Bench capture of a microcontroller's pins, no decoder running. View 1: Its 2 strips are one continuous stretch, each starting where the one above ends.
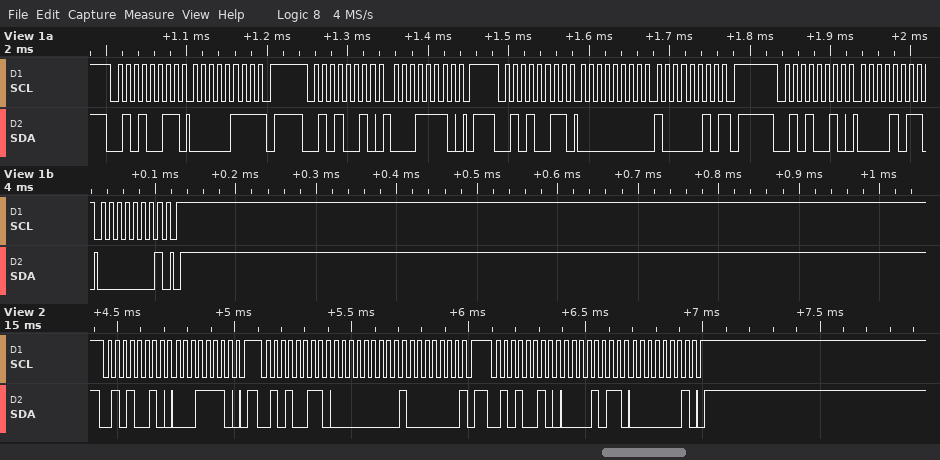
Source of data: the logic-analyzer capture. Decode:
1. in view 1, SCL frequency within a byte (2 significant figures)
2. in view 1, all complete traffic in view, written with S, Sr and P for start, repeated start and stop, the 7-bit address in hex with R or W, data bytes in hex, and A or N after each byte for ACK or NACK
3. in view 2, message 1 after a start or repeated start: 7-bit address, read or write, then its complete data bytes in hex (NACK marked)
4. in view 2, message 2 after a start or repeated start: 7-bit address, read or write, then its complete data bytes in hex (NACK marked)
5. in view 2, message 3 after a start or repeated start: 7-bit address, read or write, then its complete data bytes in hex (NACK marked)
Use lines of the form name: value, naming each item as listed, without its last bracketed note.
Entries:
in view 1, SCL frequency within a byte: 100 kHz
in view 1, all complete traffic in view, written with S, Sr and P for start, repeated start and stop, the 7-bit address in hex with R or W, data bytes in hex, and A or N after each byte for ACK or NACK: S 29R A 07 N P S 29W A 1E A P S 29R A 00 A 82 N P S 29W A 0B A 01 A P
in view 2, message 1 after a start or repeated start: 7-bit address, read or write, then its complete data bytes in hex: 0x29 write: 1E
in view 2, message 2 after a start or repeated start: 7-bit address, read or write, then its complete data bytes in hex: 0x29 read: 00 80 NACK
in view 2, message 3 after a start or repeated start: 7-bit address, read or write, then its complete data bytes in hex: 0x29 write: 0B 01
